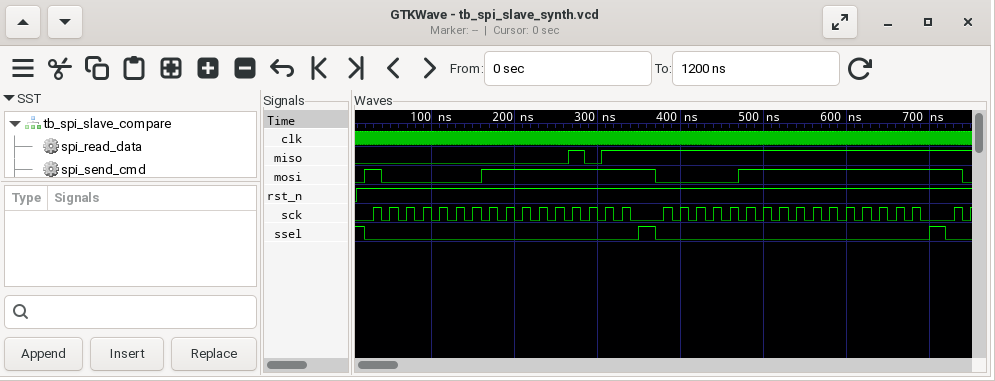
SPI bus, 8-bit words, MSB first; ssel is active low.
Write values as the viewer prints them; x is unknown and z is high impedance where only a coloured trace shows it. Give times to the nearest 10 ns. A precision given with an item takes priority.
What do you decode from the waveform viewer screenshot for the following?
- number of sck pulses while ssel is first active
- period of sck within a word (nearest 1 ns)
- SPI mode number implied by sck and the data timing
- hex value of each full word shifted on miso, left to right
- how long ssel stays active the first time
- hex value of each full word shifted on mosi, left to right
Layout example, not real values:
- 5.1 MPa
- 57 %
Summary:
- 16
- 20 ns
- 0
- 00, 0B, FF, FF
- 330 ns
- 81, FF, 07, FF
